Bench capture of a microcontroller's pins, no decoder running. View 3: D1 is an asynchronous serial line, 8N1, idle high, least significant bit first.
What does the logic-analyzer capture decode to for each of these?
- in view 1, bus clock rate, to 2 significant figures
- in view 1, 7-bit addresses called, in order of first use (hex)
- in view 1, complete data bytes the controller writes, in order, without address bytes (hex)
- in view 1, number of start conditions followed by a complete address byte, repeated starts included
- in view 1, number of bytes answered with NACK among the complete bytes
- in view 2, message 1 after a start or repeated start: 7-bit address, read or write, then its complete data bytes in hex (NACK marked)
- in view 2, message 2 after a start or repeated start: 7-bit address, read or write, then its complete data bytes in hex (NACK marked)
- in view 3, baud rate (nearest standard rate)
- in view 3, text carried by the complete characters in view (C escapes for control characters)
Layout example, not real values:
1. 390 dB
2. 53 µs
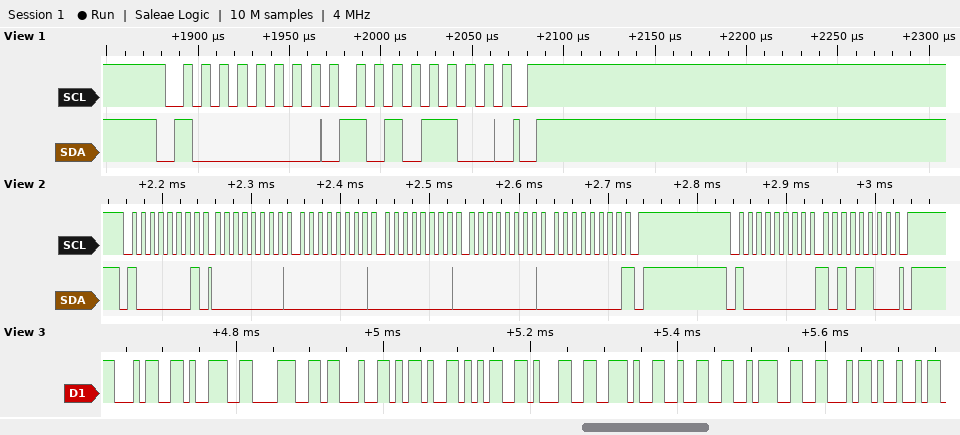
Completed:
1. 100 kHz
2. 0x40
3. AC
4. 1
5. 0
6. 0x40 read: 00 00 00 00 00 NACK
7. 0x40 write: AC
8. 115200 baud
9. "498#-51.2:FI"
